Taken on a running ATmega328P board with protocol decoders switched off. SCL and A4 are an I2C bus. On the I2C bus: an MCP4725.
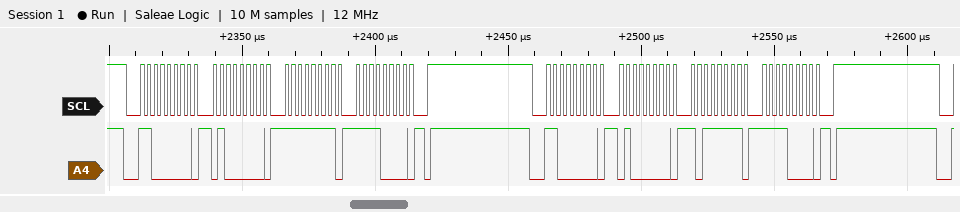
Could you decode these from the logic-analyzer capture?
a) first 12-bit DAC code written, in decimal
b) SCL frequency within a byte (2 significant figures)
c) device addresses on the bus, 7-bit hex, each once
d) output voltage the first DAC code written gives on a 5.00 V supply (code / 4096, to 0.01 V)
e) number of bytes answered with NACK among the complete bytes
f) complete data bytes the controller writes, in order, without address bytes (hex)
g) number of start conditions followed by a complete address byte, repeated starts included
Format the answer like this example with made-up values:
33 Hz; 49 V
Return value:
4095; 400 kHz; 0x60; 5.00 V; 0; 40 FF F0 40 BF F0; 2
